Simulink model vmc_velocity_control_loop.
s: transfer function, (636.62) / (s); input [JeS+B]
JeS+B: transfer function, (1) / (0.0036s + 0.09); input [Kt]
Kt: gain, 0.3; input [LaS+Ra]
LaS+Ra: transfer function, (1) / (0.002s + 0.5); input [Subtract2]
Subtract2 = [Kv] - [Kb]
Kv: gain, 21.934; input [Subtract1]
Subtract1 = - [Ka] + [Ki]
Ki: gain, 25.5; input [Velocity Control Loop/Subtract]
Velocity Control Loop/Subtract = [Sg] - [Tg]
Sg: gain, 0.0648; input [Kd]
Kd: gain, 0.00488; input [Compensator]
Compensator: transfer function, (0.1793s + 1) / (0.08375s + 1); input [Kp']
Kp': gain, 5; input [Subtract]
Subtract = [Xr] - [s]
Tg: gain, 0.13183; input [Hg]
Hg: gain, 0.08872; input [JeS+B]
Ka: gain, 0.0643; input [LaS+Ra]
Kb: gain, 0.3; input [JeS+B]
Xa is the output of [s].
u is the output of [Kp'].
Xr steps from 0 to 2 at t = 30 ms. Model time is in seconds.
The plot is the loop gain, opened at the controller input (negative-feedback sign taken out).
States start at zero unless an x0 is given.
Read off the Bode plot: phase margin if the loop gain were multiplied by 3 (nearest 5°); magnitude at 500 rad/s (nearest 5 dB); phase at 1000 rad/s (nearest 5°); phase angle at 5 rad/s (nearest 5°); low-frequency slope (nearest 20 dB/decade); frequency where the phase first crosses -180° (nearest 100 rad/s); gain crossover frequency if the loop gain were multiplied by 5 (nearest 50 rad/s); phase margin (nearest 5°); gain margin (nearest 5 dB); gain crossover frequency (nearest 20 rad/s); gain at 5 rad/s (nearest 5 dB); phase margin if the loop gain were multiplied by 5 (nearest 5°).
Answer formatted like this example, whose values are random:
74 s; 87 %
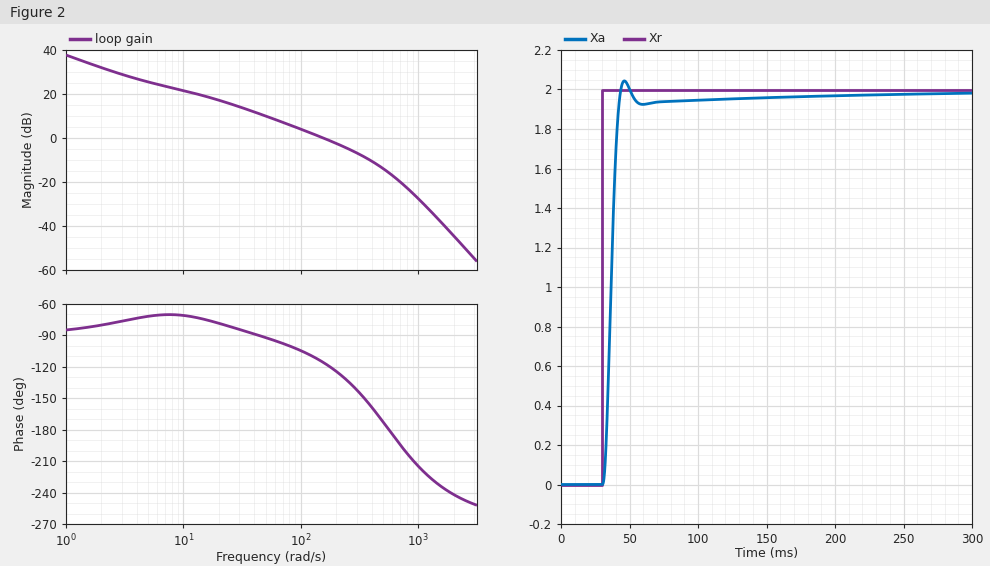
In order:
25°; -15 dB; -215°; -70°; -20 dB/decade; 600 rad/s; 500 rad/s; 65°; 15 dB; 160 rad/s; 25 dB; 5°
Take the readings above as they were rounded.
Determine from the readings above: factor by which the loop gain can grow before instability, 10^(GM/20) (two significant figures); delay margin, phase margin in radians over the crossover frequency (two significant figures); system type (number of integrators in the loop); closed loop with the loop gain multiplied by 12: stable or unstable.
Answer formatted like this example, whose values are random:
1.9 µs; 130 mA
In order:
5.6; 0.0071 s; 1; unstable
